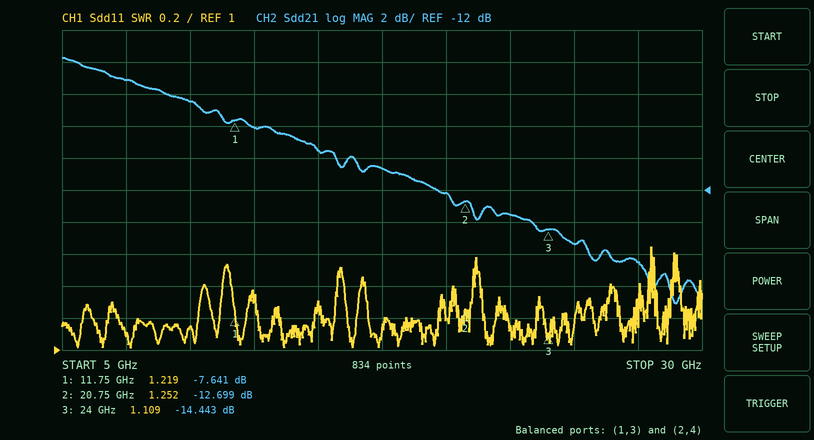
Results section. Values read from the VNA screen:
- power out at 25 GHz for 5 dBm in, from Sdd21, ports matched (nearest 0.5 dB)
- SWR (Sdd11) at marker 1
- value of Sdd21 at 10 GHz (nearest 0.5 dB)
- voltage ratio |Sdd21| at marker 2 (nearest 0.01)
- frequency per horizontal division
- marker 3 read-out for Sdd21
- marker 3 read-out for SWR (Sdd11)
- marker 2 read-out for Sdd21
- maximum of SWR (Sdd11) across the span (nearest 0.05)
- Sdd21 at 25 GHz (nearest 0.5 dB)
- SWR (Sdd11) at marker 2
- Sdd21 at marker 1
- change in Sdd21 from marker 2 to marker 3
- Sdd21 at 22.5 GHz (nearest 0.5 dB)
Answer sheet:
-10.5 dBm
1.219
-6.5 dB
0.23
2.5 GHz
-14.443 dB
1.109
-12.699 dB
1.65
-15.5 dB
1.252
-7.641 dB
-1.744 dB
-13.5 dB
